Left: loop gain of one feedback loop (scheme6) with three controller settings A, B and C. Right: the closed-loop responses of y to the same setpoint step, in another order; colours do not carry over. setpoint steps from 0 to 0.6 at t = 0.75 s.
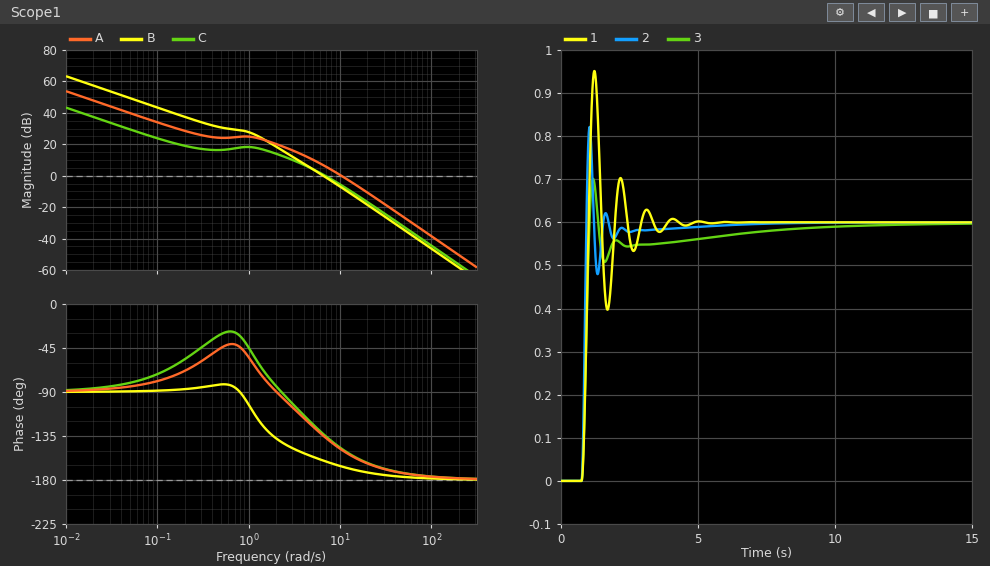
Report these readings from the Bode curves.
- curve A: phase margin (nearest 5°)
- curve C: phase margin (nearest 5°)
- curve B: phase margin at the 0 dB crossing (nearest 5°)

30°
45°
20°
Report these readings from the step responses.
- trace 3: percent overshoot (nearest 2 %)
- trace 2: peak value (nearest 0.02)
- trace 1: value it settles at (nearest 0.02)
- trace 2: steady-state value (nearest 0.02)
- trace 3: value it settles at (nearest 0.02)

16 %
0.82
0.60
0.60
0.60
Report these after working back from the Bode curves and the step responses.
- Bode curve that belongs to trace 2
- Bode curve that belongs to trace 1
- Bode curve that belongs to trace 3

A
B
C
